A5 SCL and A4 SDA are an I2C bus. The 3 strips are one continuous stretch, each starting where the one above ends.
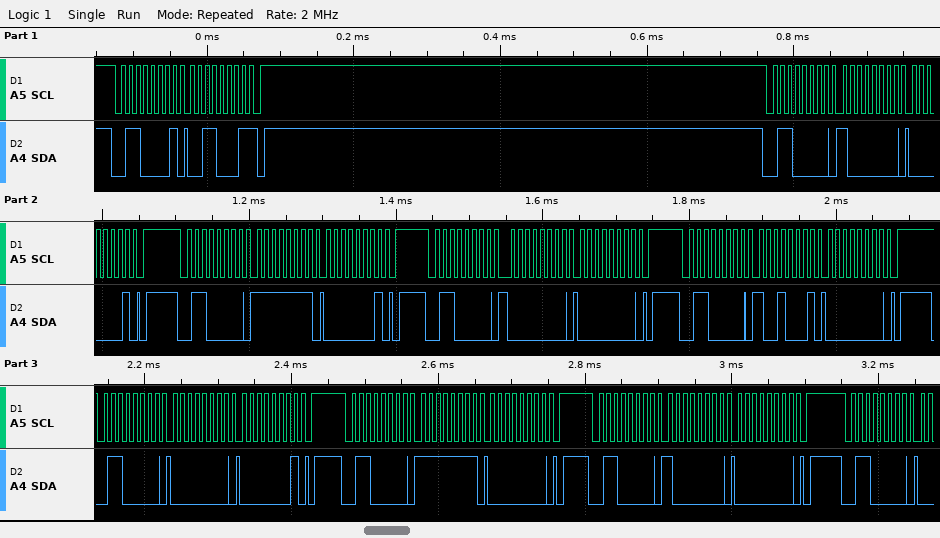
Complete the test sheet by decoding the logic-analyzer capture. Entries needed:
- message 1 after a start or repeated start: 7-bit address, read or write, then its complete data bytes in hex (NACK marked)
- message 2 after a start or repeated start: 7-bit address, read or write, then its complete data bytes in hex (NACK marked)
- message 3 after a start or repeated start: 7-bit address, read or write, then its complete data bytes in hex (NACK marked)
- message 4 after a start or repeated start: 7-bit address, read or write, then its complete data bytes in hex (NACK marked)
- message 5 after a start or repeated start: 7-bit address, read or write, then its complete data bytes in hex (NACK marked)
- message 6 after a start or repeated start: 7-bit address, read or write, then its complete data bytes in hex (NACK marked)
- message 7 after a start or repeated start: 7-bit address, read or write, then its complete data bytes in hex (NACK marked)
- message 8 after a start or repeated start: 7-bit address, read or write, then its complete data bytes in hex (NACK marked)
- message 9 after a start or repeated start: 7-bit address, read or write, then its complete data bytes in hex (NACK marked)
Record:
0x30 read: 31 NACK
0x30 write: 80 01
0x30 write: FF 01
0x30 write: 00 00
0x30 write: 91 00
0x30 write: 00 01
0x30 write: FF 00
0x30 write: 80 00
0x30 write
